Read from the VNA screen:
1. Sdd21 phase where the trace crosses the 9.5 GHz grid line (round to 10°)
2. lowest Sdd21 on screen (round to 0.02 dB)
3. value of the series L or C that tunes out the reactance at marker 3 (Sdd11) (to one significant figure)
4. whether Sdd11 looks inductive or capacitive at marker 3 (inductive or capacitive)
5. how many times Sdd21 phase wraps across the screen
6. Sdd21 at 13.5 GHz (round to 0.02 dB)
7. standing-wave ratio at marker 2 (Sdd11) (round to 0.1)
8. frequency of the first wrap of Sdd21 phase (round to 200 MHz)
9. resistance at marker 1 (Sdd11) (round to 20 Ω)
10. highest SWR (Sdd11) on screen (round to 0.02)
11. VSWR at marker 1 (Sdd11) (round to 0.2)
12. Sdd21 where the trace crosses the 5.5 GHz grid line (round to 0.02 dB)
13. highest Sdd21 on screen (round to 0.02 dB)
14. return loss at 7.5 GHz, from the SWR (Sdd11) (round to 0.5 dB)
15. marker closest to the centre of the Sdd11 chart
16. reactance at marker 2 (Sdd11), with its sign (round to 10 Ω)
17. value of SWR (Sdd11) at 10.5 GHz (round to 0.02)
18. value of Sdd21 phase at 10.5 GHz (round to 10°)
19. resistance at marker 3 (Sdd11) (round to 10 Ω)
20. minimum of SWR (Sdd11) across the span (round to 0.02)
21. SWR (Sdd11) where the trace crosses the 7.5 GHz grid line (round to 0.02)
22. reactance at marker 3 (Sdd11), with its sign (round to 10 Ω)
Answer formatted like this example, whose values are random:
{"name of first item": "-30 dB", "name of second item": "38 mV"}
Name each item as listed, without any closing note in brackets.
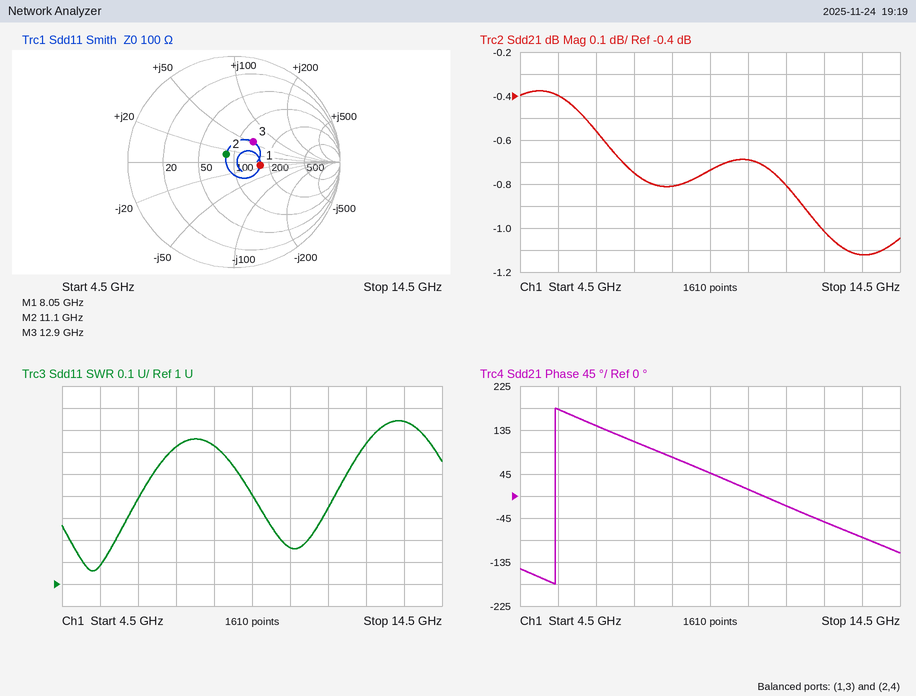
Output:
{"Sdd21 phase where the trace crosses the 9.5 GHz grid line": "50°", "lowest Sdd21 on screen": "-1.12 dB", "value of the series L or C that tunes out the reactance at marker 3 (Sdd11)": "200 fF", "whether Sdd11 looks inductive or capacitive at marker 3": "inductive", "how many times Sdd21 phase wraps across the screen": "1", "Sdd21 at 13.5 GHz": "-1.12 dB", "standing-wave ratio at marker 2 (Sdd11)": "1.2", "frequency of the first wrap of Sdd21 phase": "5.4 GHz", "resistance at marker 1 (Sdd11)": "160 Ω", "highest SWR (Sdd11) on screen": "1.74", "VSWR at marker 1 (Sdd11)": "1.6", "Sdd21 where the trace crosses the 5.5 GHz grid line": "-0.40 dB", "highest Sdd21 on screen": "-0.38 dB", "return loss at 7.5 GHz, from the SWR (Sdd11)": "12.5 dB", "marker closest to the centre of the Sdd11 chart": "marker 2", "reactance at marker 2 (Sdd11), with its sign": "+10 Ω", "value of SWR (Sdd11) at 10.5 GHz": "1.16", "value of Sdd21 phase at 10.5 GHz": "10°", "resistance at marker 3 (Sdd11)": "130 Ω", "minimum of SWR (Sdd11) across the span": "1.06", "SWR (Sdd11) where the trace crosses the 7.5 GHz grid line": "1.62", "reactance at marker 3 (Sdd11), with its sign": "+50 Ω"}
